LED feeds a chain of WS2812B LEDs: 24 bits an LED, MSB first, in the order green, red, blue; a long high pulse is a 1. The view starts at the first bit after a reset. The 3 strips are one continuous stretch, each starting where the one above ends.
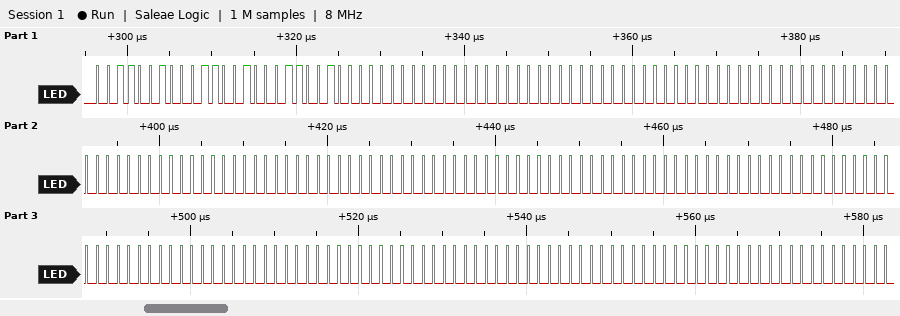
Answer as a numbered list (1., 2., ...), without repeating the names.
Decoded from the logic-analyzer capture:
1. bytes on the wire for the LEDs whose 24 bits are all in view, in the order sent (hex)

1. 32 32 32 00 00 00 00 00 00 00 00 00 00 00 00 00 00 00 00 00 00 00 00 00 00 00 00
